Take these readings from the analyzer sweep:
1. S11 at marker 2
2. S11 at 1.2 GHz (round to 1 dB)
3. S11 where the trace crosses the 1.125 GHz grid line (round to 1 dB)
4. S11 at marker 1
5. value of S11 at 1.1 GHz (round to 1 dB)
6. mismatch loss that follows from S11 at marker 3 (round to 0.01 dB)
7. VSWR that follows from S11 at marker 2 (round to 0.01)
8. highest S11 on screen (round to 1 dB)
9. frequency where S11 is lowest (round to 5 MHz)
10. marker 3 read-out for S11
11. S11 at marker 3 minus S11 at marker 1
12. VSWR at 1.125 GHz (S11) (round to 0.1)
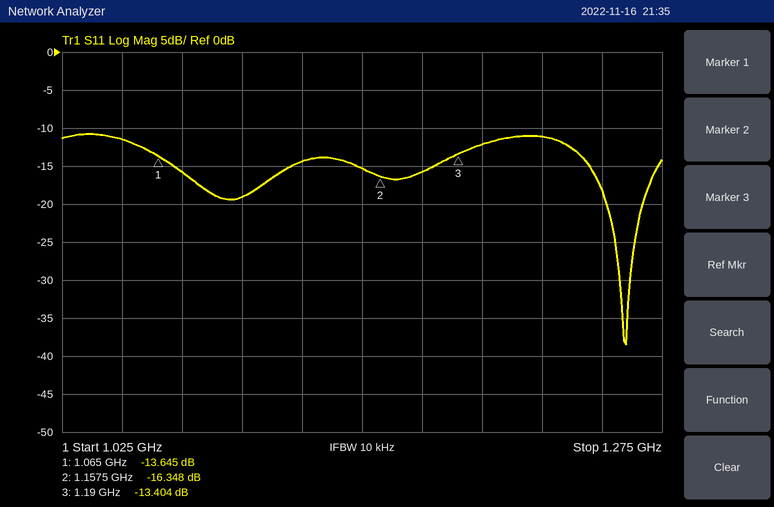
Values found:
-16.348 dB
-12 dB
-14 dB
-13.645 dB
-19 dB
0.20 dB
1.36
-11 dB
1.260 GHz
-13.404 dB
0.241 dB
1.5
